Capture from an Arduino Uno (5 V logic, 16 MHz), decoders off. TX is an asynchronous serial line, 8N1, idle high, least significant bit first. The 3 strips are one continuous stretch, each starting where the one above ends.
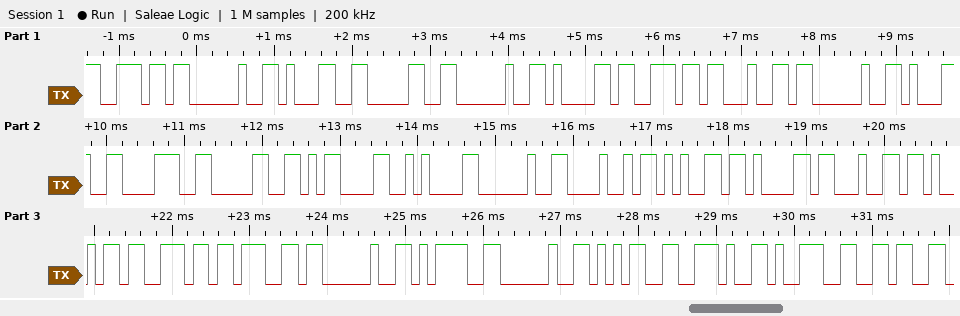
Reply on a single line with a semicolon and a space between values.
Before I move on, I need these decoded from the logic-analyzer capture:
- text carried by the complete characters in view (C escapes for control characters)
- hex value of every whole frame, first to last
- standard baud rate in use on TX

"n 10 and 180\r\n Heading = 5.96"; 6E 20 31 30 20 61 6E 64 20 31 38 30 0D 0A 20 48 65 61 64 69 6E 67 20 3D 20 35 2E 39 36; 9600 baud
